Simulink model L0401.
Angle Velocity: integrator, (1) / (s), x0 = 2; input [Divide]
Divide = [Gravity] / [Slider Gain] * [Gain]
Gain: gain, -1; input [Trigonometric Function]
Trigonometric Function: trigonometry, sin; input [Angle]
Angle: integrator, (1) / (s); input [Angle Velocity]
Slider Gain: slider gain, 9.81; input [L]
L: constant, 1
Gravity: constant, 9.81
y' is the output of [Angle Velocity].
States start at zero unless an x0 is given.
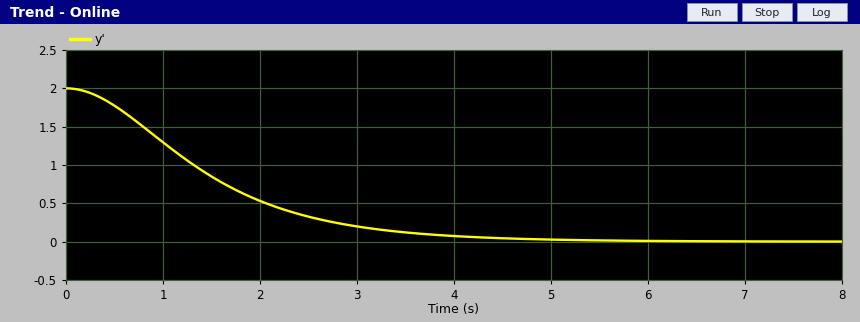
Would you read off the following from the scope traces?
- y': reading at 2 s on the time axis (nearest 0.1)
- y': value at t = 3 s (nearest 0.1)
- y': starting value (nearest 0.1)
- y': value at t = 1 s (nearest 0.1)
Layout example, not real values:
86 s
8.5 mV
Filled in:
0.5
0.2
2.0
1.3
